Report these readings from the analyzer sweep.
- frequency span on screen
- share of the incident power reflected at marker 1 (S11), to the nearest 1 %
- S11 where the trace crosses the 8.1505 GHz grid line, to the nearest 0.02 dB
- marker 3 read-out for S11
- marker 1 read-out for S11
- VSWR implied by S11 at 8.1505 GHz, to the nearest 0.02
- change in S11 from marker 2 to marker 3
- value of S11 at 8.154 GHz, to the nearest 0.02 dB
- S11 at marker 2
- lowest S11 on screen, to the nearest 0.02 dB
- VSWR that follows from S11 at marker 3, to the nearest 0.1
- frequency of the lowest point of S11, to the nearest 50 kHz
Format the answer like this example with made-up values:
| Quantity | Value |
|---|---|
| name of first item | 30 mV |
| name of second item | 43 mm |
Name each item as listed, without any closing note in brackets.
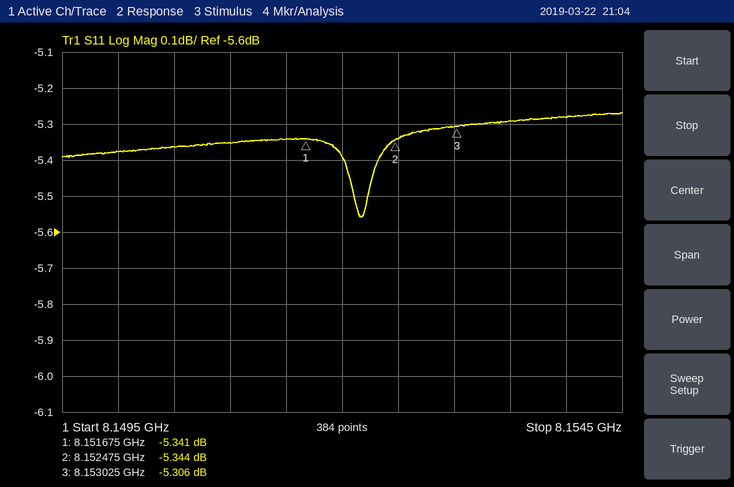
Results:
| Quantity | Value |
|---|---|
| frequency span on screen | 5 MHz |
| share of the incident power reflected at marker 1 (S11), to the nearest 1 % | 29 % |
| S11 where the trace crosses the 8.1505 GHz grid line, to the nearest 0.02 dB | -5.36 dB |
| marker 3 read-out for S11 | -5.306 dB |
| marker 1 read-out for S11 | -5.341 dB |
| VSWR implied by S11 at 8.1505 GHz, to the nearest 0.02 | 3.34 |
| change in S11 from marker 2 to marker 3 | 0.038 dB |
| value of S11 at 8.154 GHz, to the nearest 0.02 dB | -5.28 dB |
| S11 at marker 2 | -5.344 dB |
| lowest S11 on screen, to the nearest 0.02 dB | -5.56 dB |
| VSWR that follows from S11 at marker 3, to the nearest 0.1 | 3.4 |
| frequency of the lowest point of S11, to the nearest 50 kHz | 8.15215 GHz |
